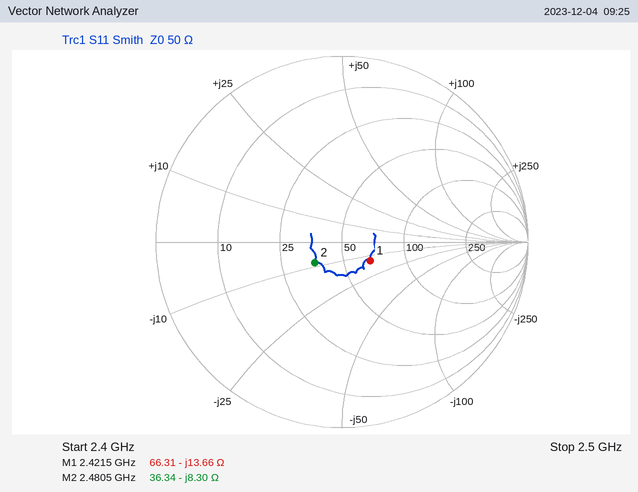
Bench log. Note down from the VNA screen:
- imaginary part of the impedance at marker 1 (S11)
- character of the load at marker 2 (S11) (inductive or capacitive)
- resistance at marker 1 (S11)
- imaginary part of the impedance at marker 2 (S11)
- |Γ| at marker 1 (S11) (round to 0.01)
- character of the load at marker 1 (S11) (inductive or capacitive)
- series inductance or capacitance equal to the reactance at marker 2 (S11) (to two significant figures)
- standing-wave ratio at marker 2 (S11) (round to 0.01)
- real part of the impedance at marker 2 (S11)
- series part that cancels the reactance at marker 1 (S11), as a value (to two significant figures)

-13.66 Ω
capacitive
66.31 Ω
-8.30 Ω
0.18
capacitive
7.7 pF
1.45
36.34 Ω
900 pH
